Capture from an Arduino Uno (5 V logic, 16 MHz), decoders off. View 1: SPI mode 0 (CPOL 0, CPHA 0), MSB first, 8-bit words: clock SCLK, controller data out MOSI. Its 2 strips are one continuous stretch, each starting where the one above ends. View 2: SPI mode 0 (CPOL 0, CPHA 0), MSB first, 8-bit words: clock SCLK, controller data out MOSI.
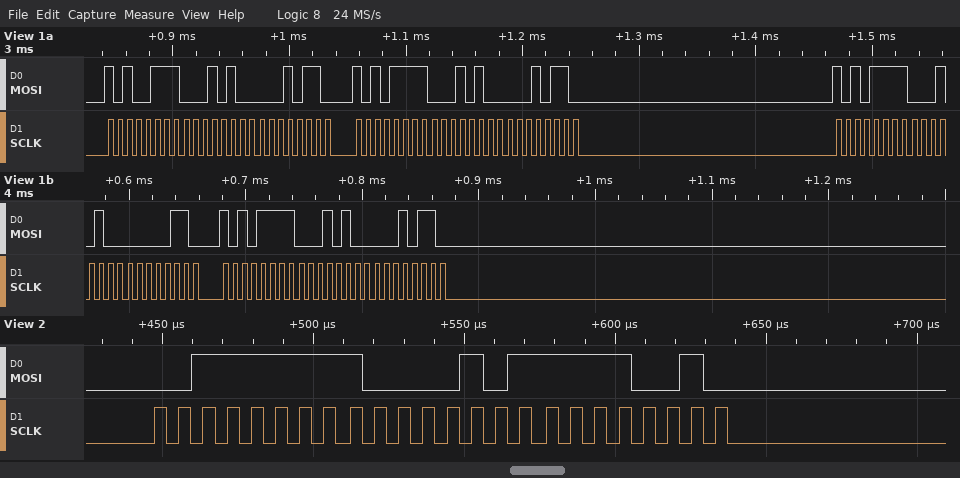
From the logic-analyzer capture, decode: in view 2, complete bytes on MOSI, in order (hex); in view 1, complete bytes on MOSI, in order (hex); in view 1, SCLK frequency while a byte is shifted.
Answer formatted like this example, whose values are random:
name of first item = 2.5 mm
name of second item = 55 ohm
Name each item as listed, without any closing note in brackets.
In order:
in view 2, complete bytes on MOSI, in order = 3F 85 F2
in view 1, complete bytes on MOSI, in order = A7 14 16 AF 14 16 AF 14 06 AF 14 16
in view 1, SCLK frequency while a byte is shifted = 125 kHz
